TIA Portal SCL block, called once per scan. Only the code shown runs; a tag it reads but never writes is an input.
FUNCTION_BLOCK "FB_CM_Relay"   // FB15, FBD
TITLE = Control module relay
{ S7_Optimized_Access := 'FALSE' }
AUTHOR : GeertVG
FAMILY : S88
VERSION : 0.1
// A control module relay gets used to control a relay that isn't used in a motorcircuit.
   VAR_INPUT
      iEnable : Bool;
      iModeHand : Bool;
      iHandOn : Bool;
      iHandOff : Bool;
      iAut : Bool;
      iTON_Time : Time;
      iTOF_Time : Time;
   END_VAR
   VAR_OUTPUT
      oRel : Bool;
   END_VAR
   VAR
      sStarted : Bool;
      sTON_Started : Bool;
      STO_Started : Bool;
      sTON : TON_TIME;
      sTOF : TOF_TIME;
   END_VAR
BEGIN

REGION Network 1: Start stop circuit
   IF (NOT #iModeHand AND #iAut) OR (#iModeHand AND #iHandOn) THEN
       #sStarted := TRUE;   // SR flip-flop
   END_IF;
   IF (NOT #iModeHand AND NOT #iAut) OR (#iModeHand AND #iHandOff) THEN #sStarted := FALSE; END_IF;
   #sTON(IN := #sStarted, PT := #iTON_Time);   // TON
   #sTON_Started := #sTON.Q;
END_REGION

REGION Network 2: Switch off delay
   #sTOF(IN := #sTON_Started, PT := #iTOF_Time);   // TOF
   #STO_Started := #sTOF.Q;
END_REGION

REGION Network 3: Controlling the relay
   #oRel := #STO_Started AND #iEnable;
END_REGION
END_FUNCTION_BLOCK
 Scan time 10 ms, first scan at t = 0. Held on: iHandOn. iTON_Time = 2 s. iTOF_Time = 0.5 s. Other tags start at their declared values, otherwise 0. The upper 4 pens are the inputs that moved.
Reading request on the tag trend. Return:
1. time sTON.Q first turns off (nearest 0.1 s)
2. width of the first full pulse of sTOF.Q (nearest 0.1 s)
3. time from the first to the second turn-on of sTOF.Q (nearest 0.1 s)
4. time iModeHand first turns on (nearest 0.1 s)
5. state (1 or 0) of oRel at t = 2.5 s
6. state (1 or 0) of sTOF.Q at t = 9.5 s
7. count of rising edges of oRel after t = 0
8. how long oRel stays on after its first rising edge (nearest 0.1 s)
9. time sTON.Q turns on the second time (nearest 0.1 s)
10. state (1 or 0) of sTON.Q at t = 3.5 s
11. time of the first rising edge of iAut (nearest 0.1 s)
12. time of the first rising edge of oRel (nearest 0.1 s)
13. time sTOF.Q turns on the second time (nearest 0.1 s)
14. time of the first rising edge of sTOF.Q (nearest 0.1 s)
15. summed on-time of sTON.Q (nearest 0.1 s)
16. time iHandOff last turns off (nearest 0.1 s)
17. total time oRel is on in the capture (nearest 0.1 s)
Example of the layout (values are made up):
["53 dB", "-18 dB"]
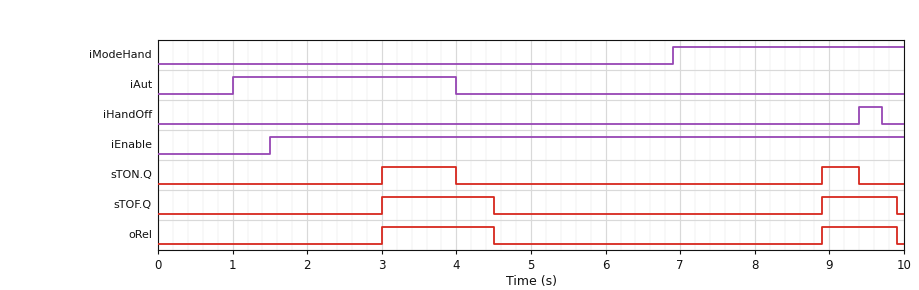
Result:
["4.0 s", "1.5 s", "5.9 s", "6.9 s", "0", "1", "2", "1.5 s", "8.9 s", "1", "1.0 s", "3.0 s", "8.9 s", "3.0 s", "1.5 s", "9.7 s", "2.5 s"]
